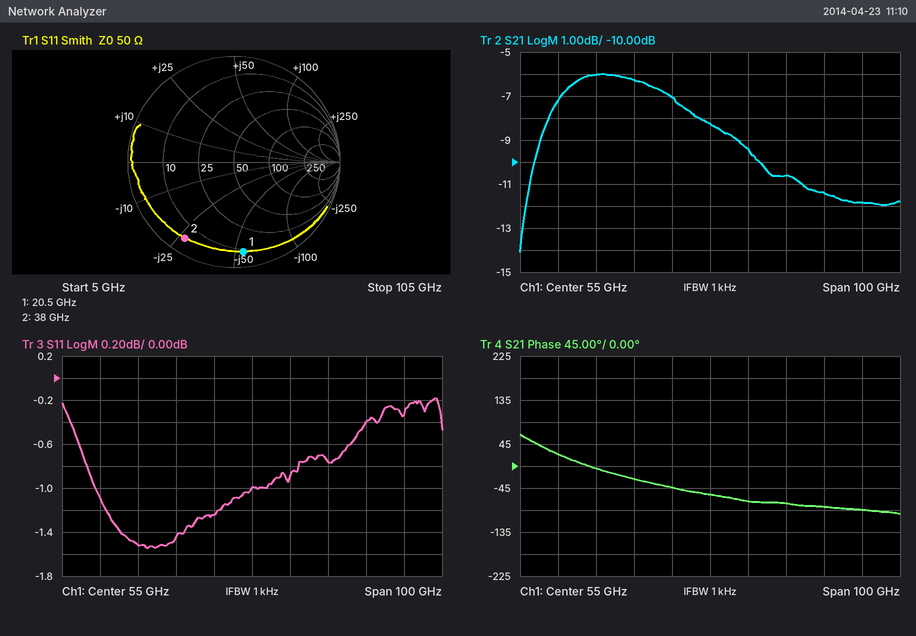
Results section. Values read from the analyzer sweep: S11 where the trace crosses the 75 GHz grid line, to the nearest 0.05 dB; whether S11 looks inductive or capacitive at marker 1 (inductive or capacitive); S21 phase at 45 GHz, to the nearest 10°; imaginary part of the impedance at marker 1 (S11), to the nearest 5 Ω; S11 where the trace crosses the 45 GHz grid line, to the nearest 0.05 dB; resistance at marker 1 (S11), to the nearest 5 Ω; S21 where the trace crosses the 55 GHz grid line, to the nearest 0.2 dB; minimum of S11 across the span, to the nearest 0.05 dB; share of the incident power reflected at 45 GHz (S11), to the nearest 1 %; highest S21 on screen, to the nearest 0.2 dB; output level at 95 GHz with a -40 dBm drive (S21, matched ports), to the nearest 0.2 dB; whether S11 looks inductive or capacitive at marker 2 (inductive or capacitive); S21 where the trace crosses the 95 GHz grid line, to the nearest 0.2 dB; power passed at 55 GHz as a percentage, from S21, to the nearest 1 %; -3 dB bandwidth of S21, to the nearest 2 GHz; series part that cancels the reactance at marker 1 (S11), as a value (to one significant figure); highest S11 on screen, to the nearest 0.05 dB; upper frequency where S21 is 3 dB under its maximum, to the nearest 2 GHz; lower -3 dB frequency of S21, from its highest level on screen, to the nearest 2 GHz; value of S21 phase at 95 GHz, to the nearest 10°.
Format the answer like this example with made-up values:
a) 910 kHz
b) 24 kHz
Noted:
a) -0.75 dB
b) capacitive
c) -40°
d) -55 Ω
e) -1.25 dB
f) 10 Ω
g) -8.2 dB
h) -1.55 dB
i) 75 %
j) -6.0 dB
k) -51.8 dBm
l) capacitive
m) -11.8 dB
n) 15 %
o) 52 GHz
p) 400 pH
q) -0.20 dB
r) 62 GHz
s) 10 GHz
t) -90°
